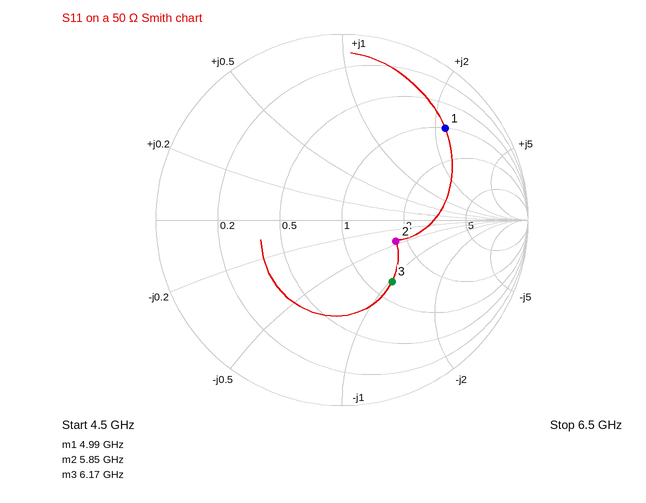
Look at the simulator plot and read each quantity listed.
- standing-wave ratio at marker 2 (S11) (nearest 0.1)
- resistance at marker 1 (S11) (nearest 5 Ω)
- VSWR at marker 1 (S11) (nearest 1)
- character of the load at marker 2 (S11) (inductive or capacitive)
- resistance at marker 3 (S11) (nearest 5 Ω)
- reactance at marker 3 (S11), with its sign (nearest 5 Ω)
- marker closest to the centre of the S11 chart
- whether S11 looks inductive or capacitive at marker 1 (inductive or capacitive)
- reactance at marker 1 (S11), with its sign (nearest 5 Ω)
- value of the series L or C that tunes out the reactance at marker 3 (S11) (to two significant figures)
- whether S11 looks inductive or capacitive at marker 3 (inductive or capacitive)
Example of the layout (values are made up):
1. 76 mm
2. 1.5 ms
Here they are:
1. 1.9
2. 50 Ω
3. 7
4. capacitive
5. 65 Ω
6. -50 Ω
7. marker 2
8. inductive
9. +110 Ω
10. 1.3 nH
11. capacitive
